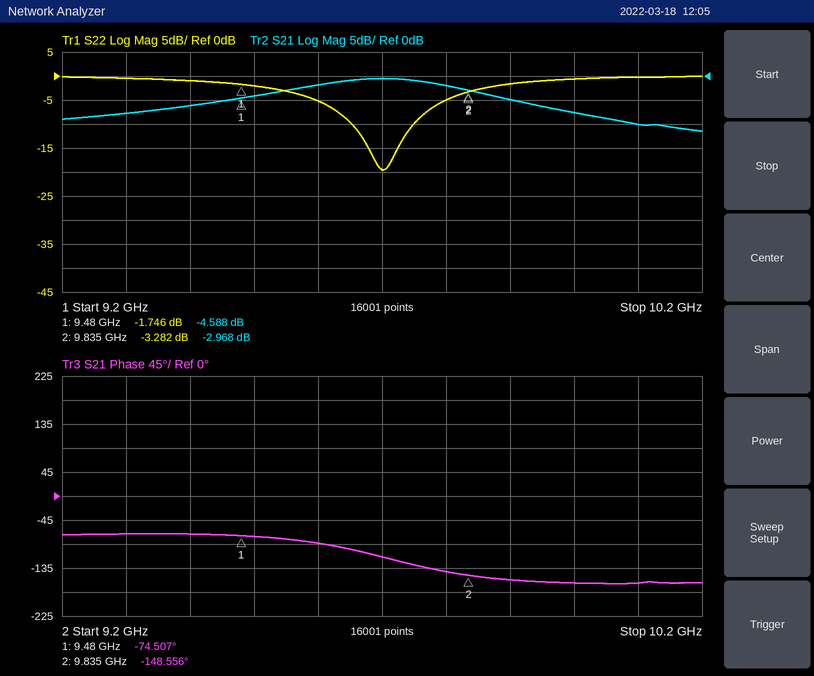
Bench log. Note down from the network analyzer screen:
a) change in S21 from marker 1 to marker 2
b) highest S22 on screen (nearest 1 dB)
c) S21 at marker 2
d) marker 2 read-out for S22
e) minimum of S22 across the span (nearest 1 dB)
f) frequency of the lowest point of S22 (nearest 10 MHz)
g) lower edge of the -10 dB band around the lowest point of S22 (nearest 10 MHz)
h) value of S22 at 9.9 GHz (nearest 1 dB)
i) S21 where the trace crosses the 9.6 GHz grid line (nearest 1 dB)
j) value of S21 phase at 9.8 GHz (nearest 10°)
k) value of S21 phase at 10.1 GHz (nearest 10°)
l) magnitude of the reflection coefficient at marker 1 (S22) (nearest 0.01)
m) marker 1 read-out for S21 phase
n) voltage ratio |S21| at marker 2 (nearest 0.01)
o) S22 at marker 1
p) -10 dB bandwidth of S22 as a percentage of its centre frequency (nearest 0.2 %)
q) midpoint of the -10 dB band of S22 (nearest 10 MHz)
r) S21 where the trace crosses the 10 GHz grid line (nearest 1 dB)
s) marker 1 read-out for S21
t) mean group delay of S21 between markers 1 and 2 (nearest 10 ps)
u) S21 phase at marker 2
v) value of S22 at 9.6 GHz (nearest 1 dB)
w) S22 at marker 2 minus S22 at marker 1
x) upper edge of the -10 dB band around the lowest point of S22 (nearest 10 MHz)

1.620 dB
0 dB
-2.968 dB
-3.282 dB
-20 dB
9.70 GHz
9.65 GHz
-2 dB
-2 dB
-140°
-160°
0.82
-74.507°
0.71
-1.746 dB
1.0 %
9.70 GHz
-8 dB
-4.588 dB
580 ps
-148.556°
-5 dB
-1.536 dB
9.75 GHz
